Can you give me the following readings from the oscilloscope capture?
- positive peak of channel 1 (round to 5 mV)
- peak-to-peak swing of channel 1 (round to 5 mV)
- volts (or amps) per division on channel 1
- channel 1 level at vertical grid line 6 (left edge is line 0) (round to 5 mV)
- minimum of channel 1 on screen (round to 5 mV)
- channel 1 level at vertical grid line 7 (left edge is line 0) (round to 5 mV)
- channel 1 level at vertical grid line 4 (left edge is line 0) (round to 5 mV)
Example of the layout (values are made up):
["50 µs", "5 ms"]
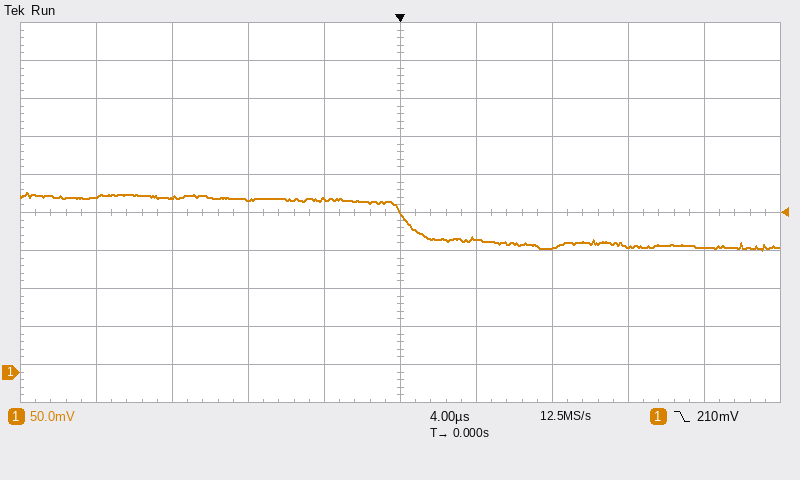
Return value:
["235 mV", "75 mV", "50 mV", "175 mV", "160 mV", "165 mV", "225 mV"]
